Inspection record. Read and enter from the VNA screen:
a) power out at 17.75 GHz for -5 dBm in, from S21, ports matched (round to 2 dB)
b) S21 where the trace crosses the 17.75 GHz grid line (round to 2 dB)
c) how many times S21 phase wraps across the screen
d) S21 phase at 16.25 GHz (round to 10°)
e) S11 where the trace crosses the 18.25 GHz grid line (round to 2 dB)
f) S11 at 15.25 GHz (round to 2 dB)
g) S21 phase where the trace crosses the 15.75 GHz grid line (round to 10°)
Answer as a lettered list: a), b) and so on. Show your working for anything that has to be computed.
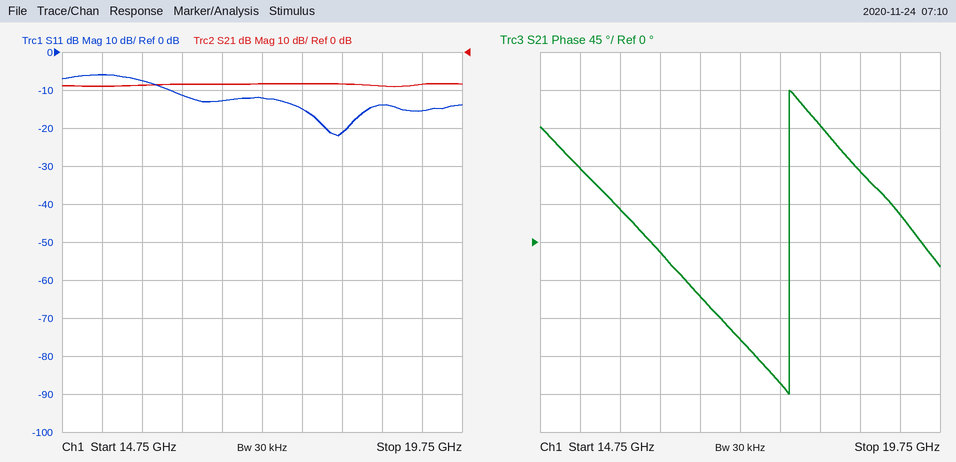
a) -5 dBm + (-8 dB) = -14 dBm
b) -8 dB
c) 1
d) -10°
e) -22 dB
f) -6 dB
g) 40°
